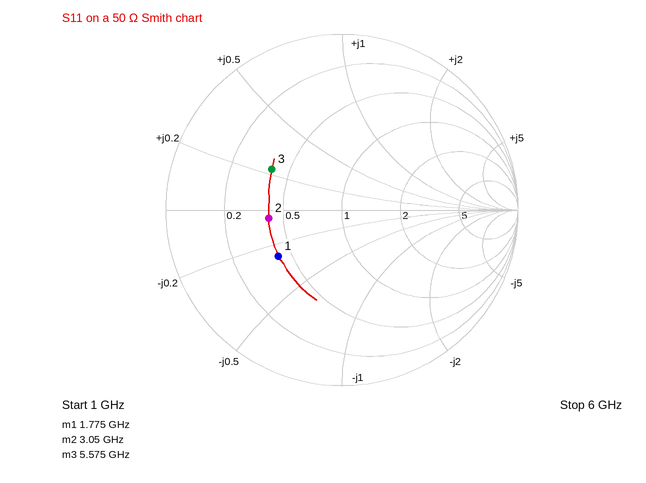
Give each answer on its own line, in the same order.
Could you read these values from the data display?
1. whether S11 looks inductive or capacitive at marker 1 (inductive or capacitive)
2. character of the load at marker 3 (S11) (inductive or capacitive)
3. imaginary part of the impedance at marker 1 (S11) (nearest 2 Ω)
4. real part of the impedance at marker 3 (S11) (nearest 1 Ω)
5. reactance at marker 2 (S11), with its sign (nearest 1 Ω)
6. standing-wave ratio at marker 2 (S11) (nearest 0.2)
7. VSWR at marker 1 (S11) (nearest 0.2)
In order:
capacitive
inductive
-14 Ω
20 Ω
-2 Ω
2.4
2.6
